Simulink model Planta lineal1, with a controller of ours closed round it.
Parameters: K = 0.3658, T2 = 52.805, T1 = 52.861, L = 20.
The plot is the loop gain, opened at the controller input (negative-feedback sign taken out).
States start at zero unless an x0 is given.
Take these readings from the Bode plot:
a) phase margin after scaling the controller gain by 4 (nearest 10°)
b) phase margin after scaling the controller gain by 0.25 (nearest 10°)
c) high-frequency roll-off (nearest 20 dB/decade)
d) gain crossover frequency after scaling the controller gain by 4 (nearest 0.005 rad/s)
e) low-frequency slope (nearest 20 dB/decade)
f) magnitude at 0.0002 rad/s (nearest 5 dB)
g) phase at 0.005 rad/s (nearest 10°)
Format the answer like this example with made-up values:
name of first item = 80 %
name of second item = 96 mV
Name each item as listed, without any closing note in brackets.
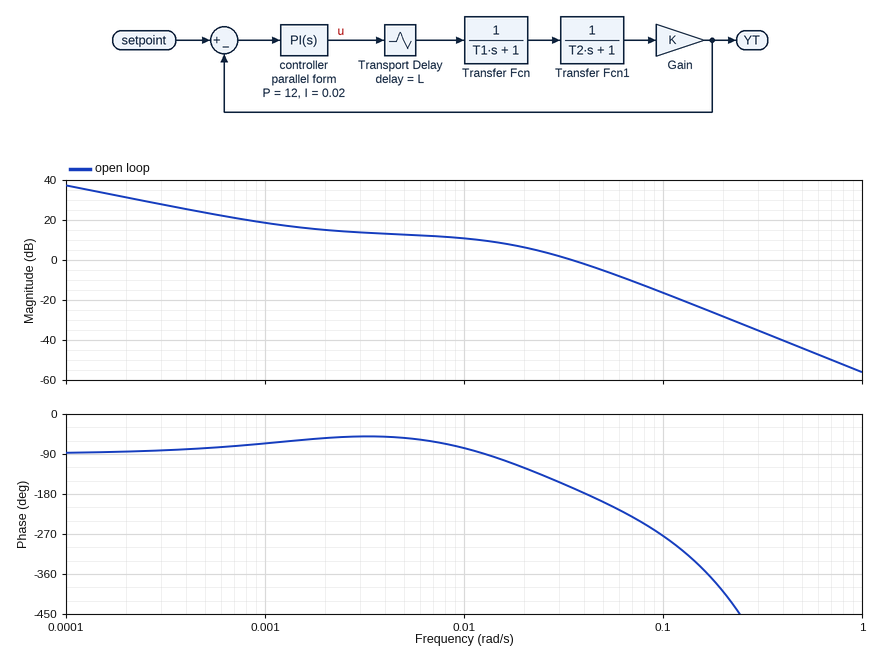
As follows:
phase margin after scaling the controller gain by 4 = -60°
phase margin after scaling the controller gain by 0.25 = 120°
high-frequency roll-off = -40 dB/decade
gain crossover frequency after scaling the controller gain by 4 = 0.075 rad/s
low-frequency slope = -20 dB/decade
magnitude at 0.0002 rad/s = 30 dB
phase at 0.005 rad/s = -50°
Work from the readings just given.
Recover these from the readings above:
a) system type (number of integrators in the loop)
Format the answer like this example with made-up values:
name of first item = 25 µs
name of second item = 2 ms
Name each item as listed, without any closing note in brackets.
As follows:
system type = 1
